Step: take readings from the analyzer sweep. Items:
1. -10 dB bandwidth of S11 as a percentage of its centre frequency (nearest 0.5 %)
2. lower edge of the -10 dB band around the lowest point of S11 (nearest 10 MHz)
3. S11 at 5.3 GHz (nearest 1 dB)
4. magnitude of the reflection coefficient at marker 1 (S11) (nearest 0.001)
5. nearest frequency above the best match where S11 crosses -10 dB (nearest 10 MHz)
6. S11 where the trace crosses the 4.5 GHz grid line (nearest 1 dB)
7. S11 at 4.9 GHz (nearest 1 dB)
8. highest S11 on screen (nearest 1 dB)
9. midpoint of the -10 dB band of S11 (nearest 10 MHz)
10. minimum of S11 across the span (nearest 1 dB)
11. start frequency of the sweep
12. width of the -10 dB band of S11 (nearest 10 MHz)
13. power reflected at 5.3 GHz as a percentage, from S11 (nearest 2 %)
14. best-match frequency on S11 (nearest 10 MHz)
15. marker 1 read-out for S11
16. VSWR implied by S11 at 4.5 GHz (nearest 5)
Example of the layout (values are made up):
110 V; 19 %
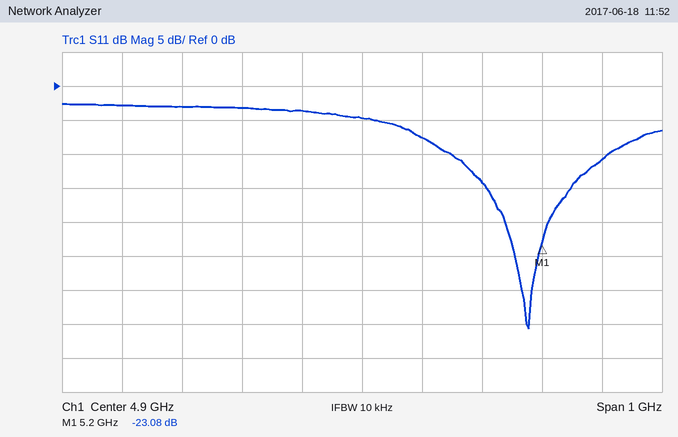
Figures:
5.0 %; 5.05 GHz; -11 dB; 0.070; 5.31 GHz; -3 dB; -5 dB; -3 dB; 5.18 GHz; -36 dB; 4.4 GHz; 260 MHz; 8 %; 5.18 GHz; -23.08 dB; 5
